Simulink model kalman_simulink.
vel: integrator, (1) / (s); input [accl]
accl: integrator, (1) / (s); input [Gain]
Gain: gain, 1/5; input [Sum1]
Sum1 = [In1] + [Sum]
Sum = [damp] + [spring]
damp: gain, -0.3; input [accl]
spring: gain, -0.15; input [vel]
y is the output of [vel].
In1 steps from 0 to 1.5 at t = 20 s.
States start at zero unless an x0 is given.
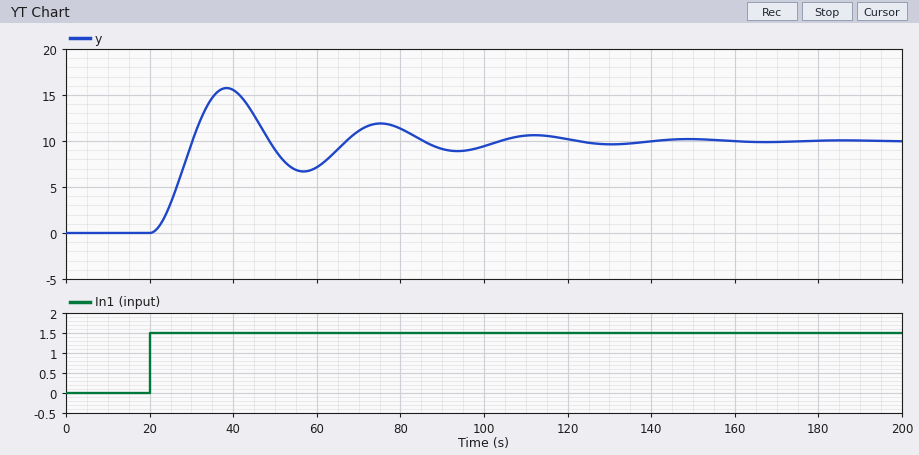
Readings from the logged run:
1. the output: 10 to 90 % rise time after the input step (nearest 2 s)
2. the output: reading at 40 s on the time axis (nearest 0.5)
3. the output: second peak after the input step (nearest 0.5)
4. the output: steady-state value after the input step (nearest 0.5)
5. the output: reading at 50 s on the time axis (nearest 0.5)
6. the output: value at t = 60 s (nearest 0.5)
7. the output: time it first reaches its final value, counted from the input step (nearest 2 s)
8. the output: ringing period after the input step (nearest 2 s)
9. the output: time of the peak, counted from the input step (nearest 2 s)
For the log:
6 s
15.5
12.0
10.0
9.0
7.0
10 s
36 s
18 s
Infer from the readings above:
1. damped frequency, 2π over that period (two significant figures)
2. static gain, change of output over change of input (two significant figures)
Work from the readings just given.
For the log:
0.17 rad/s
6.7
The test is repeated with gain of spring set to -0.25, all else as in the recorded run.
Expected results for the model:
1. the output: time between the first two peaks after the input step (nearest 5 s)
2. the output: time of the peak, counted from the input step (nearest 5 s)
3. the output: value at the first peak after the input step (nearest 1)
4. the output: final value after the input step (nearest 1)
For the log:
30 s
15 s
10
6
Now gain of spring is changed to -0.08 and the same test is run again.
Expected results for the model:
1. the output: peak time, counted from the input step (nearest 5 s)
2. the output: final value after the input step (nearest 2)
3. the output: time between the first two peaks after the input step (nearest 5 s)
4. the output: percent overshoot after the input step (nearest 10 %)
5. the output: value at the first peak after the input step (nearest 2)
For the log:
25 s
18
50 s
50 %
28
